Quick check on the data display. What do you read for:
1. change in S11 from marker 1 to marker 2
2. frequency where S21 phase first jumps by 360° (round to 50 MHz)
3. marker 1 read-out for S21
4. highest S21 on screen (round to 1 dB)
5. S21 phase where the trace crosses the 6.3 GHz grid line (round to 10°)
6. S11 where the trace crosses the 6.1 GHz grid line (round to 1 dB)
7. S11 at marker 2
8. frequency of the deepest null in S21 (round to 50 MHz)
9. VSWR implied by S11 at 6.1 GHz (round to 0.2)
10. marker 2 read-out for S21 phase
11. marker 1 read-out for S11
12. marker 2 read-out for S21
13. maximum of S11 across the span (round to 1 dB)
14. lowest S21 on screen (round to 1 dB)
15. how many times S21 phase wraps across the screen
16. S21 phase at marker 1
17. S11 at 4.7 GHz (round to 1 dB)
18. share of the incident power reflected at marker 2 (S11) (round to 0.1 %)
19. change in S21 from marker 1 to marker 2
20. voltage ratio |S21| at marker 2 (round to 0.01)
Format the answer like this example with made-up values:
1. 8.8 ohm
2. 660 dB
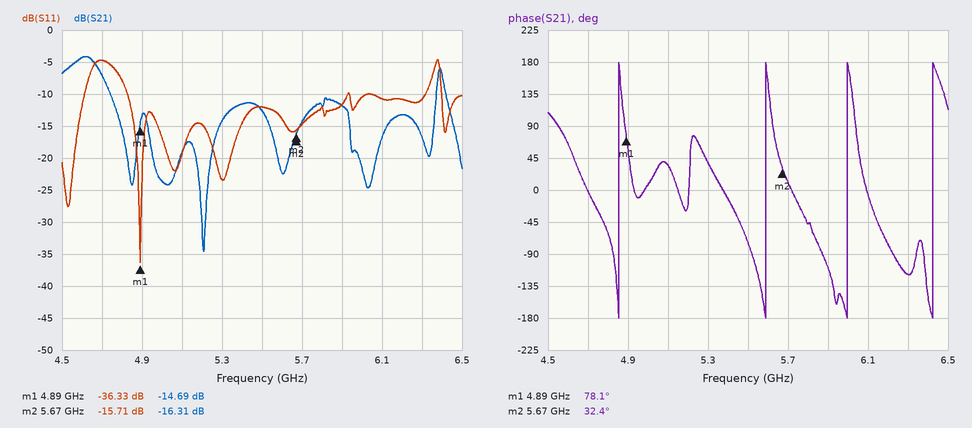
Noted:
1. 20.62 dB
2. 4.85 GHz
3. -14.69 dB
4. -4 dB
5. -120°
6. -11 dB
7. -15.71 dB
8. 5.20 GHz
9. 1.8
10. 32.4°
11. -36.33 dB
12. -16.31 dB
13. -5 dB
14. -35 dB
15. 4
16. 78.1°
17. -5 dB
18. 2.7 %
19. -1.62 dB
20. 0.15
